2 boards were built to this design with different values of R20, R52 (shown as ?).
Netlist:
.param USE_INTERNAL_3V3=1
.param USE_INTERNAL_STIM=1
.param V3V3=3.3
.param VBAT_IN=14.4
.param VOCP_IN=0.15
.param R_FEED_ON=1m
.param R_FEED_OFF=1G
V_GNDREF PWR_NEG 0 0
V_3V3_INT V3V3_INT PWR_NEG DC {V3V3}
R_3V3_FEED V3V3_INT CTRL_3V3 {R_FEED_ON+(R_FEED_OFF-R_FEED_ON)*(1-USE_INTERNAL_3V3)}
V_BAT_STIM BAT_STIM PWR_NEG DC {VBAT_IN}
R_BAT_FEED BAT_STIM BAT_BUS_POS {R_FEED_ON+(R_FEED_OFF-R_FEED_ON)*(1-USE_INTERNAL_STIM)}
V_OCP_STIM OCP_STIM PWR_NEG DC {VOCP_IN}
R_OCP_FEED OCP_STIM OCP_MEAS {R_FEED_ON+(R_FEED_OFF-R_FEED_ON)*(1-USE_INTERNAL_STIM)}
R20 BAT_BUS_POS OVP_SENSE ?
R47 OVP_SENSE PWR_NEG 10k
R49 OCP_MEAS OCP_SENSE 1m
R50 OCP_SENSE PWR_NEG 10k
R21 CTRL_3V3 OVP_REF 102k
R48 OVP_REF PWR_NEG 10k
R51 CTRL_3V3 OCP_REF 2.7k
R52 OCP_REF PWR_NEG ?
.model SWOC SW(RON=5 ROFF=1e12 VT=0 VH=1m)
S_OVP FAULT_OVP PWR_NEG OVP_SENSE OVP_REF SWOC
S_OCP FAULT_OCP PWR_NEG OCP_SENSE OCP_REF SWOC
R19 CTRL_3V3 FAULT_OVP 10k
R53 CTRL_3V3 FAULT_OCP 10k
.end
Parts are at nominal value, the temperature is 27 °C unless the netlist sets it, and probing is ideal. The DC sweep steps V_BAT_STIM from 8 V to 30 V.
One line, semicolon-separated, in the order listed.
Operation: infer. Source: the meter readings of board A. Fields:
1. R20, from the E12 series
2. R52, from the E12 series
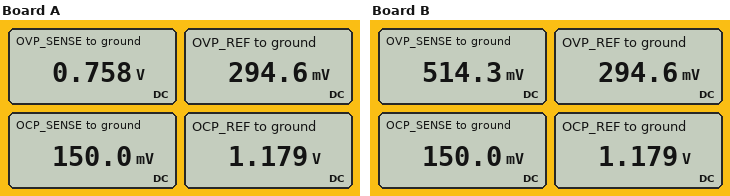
180 kΩ; 1.5 kΩ
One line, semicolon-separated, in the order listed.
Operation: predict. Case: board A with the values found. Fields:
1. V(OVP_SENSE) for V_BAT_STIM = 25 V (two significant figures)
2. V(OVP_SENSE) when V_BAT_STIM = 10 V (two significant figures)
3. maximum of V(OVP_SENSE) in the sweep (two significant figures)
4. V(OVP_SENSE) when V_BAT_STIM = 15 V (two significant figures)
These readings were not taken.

1.3 V; 530 mV; 1.6 V; 790 mV
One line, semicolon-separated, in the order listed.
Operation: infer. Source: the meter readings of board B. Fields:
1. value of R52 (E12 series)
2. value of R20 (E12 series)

1.5 kΩ; 270 kΩ
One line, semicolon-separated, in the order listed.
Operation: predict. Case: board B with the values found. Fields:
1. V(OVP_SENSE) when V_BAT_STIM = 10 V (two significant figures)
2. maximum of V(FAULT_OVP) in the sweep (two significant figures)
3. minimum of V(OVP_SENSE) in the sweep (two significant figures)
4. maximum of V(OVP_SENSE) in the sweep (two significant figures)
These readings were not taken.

360 mV; 3.3 V; 290 mV; 1.1 V
